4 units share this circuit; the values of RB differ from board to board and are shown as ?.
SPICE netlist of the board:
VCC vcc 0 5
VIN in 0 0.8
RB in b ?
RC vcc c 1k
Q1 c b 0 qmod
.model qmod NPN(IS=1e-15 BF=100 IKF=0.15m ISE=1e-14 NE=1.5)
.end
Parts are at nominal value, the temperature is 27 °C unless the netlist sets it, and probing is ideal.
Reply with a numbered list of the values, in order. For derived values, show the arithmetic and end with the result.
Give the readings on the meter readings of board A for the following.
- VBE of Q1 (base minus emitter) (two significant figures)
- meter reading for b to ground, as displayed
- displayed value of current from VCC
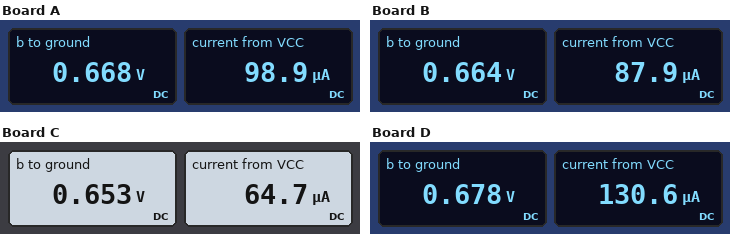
1. 668 mV = 670 mV
2. 0.668 V
3. 98.9 µA
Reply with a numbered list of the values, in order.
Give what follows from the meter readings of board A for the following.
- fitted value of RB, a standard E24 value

1. 68 kΩ
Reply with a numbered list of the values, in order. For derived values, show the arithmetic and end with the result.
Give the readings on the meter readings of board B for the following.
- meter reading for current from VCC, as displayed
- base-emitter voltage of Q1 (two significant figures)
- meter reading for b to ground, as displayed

1. 87.9 µA
2. 664 mV = 660 mV
3. 0.664 V
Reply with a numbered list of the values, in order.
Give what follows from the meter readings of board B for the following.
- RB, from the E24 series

1. 82 kΩ
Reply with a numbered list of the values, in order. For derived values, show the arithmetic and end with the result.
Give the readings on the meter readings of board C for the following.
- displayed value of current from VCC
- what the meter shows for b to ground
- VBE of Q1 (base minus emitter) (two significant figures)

1. 64.7 µA
2. 0.653 V
3. 653 mV = 650 mV
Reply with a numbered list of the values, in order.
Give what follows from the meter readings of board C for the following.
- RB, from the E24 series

1. 130 kΩ
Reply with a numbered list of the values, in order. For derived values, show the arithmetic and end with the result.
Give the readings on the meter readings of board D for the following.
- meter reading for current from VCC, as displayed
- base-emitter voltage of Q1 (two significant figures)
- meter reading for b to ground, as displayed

1. 130.6 µA
2. 678 mV = 680 mV
3. 0.678 V
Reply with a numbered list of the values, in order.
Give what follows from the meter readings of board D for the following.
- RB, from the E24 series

1. 43 kΩ
